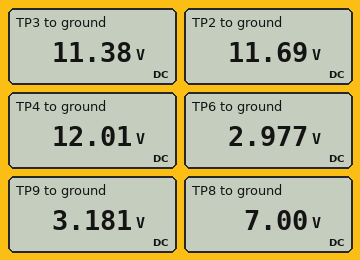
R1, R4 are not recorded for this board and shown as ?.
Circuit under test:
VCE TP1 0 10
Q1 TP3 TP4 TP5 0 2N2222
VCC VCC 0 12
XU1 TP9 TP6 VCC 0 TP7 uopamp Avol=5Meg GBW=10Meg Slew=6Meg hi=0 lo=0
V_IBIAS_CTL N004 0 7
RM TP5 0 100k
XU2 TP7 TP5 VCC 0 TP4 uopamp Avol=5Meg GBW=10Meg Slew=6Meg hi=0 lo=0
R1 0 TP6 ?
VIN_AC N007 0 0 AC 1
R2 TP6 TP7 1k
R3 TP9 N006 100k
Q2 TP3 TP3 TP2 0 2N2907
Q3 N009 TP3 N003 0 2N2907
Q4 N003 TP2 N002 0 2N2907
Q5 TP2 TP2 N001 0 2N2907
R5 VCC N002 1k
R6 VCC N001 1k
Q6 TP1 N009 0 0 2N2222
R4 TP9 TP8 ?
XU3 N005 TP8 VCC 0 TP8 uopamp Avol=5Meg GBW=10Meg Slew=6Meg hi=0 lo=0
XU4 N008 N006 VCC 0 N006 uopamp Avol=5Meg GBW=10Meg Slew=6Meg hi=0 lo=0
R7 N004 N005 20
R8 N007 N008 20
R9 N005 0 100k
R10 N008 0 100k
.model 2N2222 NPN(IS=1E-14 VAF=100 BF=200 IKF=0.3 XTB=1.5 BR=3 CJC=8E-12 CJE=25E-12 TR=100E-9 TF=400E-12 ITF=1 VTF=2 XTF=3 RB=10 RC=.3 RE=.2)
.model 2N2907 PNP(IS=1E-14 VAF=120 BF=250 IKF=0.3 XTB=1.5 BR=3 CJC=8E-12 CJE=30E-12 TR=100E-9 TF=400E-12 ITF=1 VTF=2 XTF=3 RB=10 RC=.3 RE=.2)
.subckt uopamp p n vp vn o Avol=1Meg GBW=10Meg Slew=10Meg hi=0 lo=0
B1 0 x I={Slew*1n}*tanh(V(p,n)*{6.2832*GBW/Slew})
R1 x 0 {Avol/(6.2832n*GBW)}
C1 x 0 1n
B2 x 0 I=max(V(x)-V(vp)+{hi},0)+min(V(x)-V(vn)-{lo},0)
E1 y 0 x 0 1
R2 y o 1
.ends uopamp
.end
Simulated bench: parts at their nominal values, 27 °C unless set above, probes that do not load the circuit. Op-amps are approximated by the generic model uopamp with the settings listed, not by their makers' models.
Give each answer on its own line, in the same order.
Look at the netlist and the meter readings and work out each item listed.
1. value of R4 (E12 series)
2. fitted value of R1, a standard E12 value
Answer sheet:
120 kΩ
330 Ω
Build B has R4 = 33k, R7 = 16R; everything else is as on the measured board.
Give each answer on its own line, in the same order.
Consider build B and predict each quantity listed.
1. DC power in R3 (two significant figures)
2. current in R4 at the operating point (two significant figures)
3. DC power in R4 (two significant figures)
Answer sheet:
280 µW
53 µA
91 µW
